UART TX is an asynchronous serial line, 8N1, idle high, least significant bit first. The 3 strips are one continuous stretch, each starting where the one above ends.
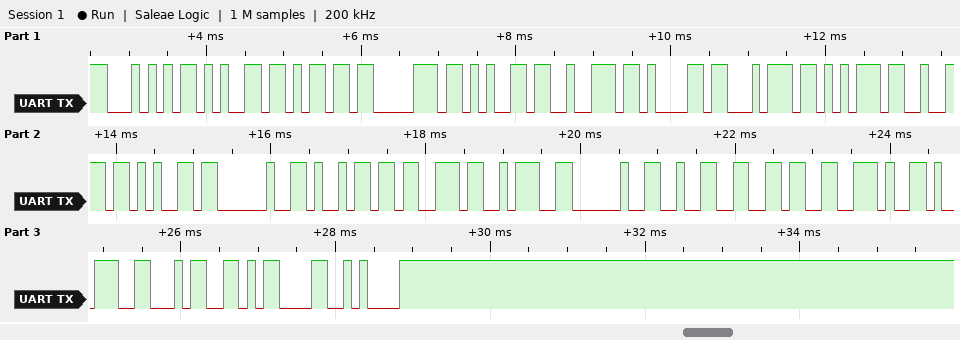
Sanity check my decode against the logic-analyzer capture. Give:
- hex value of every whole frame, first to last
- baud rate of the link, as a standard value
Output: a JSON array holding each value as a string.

["54 65 6D 70 65 72 61 74 75 72 65 20 69 73 3A 20 32 36 2E 39 34 0D 0A", "9600 baud"]
